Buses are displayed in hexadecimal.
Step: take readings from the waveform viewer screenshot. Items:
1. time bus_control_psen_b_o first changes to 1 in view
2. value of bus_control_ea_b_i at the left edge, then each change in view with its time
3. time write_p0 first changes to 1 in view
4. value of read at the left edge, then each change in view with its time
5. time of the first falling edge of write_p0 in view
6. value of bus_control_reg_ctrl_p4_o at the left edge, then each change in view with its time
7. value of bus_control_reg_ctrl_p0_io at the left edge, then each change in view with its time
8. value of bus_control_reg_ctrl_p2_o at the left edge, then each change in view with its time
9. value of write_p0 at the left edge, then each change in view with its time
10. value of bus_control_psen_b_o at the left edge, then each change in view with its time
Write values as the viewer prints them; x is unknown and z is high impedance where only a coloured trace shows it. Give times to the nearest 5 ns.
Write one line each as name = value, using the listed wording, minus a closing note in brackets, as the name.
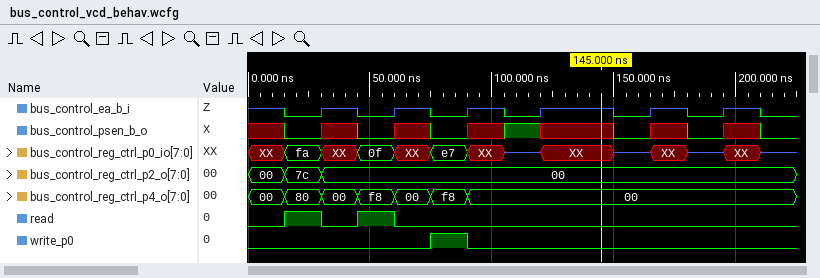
time bus_control_psen_b_o first changes to 1 in view = 105 ns
value of bus_control_ea_b_i at the left edge, then each change in view with its time = z, 0 at 15 ns, z at 30 ns, 0 at 45 ns, z at 60 ns, 0 at 75 ns, z at 90 ns, 0 at 105 ns, z at 120 ns, 0 at 150 ns, z at 165 ns, 0 at 180 ns, z at 195 ns, 0 at 210 ns
time write_p0 first changes to 1 in view = 75 ns
value of read at the left edge, then each change in view with its time = 0, 1 at 15 ns, 0 at 30 ns, 1 at 45 ns, 0 at 60 ns
time of the first falling edge of write_p0 in view = 90 ns
value of bus_control_reg_ctrl_p4_o at the left edge, then each change in view with its time = 00, 80 at 15 ns, 00 at 30 ns, f8 at 45 ns, 00 at 60 ns, f8 at 75 ns, 00 at 90 ns
value of bus_control_reg_ctrl_p0_io at the left edge, then each change in view with its time = XX, fa at 15 ns, XX at 30 ns, 0f at 45 ns, XX at 60 ns, e7 at 75 ns, XX at 90 ns, z at 105 ns, XX at 120 ns, z at 150 ns, XX at 165 ns, z at 180 ns, XX at 195 ns, z at 210 ns
value of bus_control_reg_ctrl_p2_o at the left edge, then each change in view with its time = 00, 7c at 15 ns, 00 at 30 ns
value of write_p0 at the left edge, then each change in view with its time = 0, 1 at 75 ns, 0 at 90 ns
value of bus_control_psen_b_o at the left edge, then each change in view with its time = x, 0 at 15 ns, x at 30 ns, 0 at 45 ns, x at 60 ns, 0 at 75 ns, x at 90 ns, 1 at 105 ns, x at 120 ns, 0 at 150 ns, x at 165 ns, 0 at 180 ns, x at 195 ns, 0 at 210 ns
